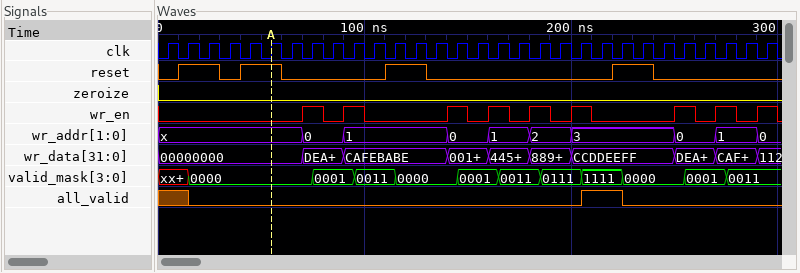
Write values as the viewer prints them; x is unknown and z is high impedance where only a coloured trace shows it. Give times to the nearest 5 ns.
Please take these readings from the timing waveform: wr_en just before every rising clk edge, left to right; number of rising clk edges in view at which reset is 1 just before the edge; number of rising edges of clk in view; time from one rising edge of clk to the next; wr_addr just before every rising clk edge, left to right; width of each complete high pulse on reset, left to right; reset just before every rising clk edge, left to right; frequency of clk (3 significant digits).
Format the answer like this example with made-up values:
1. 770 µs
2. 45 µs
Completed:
1. 0 0 0 0 0 0 0 1 0 1 0 0 0 0 1 0 1 0 1 0 1 0 0 0 0 1 0 1 0 1
2. 8
3. 30
4. 10 ns
5. x, x, x, x, x, x, x, 0, 0, 1, 1, 1, 1, 1, 0, 0, 1, 1, 2, 2, 3, 3, 3, 3, 3, 0, 0, 1, 1, 0
6. 20 ns, 20 ns, 20 ns, 20 ns
7. 0 1 1 0 1 1 0 0 0 0 0 1 1 0 0 0 0 0 0 0 0 0 1 1 0 0 0 0 0 0
8. 100 MHz
